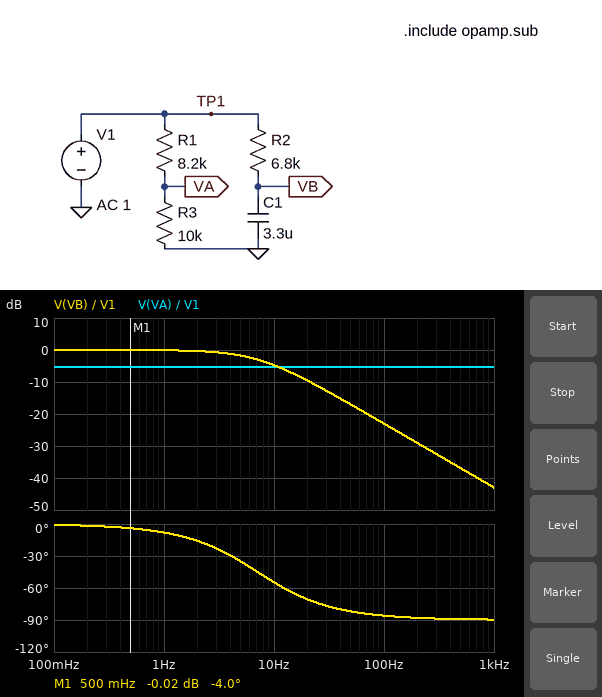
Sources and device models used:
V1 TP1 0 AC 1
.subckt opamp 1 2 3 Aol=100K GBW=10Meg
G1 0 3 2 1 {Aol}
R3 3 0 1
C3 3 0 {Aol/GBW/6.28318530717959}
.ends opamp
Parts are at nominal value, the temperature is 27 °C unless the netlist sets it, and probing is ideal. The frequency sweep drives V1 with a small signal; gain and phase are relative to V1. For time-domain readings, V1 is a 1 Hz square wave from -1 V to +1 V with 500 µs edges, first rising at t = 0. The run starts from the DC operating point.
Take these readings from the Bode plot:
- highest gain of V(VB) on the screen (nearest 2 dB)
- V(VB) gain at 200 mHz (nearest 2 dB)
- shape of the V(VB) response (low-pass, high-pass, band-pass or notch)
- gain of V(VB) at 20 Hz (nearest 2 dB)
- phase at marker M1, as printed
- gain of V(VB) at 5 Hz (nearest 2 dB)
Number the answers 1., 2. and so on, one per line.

1. 0 dB
2. 0 dB
3. low-pass
4. -10 dB
5. -4.0 deg
6. -2 dB
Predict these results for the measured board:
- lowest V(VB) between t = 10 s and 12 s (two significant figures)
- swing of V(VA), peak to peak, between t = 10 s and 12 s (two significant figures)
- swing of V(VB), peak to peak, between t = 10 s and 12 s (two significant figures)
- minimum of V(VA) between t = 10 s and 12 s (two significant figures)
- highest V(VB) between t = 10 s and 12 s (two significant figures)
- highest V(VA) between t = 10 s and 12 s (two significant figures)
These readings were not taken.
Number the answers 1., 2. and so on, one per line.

1. -1.0 V
2. 1.1 V
3. 2.0 V
4. -550 mV
5. 1.0 V
6. 550 mV
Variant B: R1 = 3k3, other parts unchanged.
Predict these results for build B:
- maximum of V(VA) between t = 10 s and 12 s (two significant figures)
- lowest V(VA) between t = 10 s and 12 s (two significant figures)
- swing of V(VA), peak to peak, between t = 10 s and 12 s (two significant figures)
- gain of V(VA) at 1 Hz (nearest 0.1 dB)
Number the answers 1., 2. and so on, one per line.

1. 750 mV
2. -750 mV
3. 1.5 V
4. -2.5 dB
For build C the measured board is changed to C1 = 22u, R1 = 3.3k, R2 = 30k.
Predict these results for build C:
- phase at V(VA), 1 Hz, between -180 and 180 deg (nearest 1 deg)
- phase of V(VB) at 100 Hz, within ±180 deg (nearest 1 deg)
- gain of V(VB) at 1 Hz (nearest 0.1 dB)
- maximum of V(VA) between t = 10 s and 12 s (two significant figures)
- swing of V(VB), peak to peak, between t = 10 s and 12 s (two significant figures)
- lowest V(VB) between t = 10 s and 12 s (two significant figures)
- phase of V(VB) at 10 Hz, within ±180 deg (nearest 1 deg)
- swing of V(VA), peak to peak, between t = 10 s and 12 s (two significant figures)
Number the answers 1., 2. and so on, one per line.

1. 0 deg
2. -90 deg
3. -12.6 dB
4. 750 mV
5. 720 mV
6. -360 mV
7. -89 deg
8. 1.5 V
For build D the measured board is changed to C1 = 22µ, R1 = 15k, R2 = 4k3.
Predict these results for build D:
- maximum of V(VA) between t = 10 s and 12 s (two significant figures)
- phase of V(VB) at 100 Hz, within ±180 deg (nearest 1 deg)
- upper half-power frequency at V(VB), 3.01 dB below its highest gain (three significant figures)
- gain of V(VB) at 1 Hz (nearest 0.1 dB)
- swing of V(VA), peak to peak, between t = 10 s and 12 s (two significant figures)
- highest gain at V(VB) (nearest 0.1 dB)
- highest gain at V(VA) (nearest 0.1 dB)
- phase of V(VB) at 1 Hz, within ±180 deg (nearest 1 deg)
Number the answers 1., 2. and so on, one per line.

1. 400 mV
2. -89 deg
3. 1.68 Hz
4. -1.3 dB
5. 800 mV
6. 0 dB
7. -8.0 dB
8. -31 deg
